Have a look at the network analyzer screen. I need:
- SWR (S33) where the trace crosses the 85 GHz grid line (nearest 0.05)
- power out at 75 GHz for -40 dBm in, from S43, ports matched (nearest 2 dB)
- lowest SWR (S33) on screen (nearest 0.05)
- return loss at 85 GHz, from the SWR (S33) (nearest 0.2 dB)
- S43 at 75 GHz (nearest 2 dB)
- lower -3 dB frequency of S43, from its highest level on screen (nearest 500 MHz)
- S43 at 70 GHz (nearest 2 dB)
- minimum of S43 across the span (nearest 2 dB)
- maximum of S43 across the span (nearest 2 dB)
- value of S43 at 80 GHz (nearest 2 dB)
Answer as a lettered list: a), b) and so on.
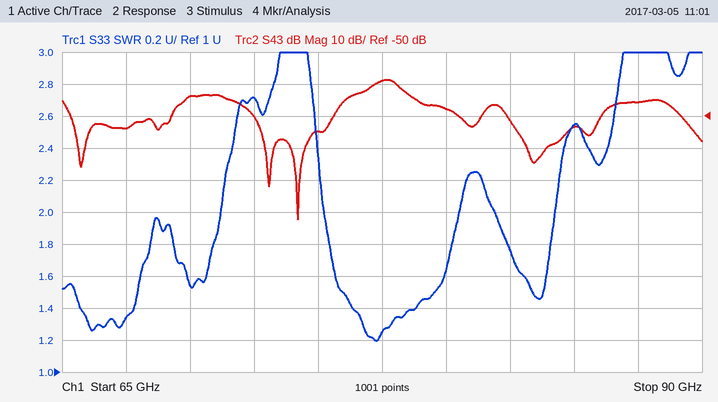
a) 2.55
b) -94 dBm
c) 1.20
d) 7.2 dB
e) -54 dB
f) 77.0 GHz
g) -44 dB
h) -82 dB
i) -38 dB
j) -48 dB
